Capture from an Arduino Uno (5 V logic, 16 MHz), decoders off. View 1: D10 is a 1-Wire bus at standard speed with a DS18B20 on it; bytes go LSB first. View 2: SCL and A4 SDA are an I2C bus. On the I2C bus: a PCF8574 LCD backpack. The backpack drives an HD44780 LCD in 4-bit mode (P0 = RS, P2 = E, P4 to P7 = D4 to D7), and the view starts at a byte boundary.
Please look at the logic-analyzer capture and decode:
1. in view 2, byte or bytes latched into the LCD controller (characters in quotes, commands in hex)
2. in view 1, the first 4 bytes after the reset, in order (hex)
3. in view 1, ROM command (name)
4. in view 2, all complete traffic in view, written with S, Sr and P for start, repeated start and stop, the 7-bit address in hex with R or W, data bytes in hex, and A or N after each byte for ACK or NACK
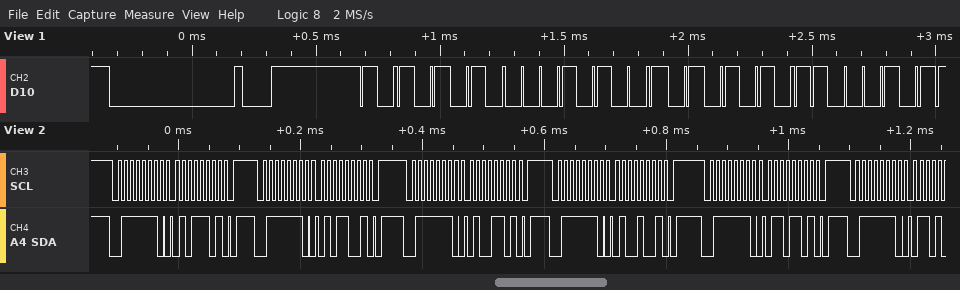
'T'
55 28 55 A3
Match ROM
S 3FW A 5D A P S 3FW A 59 A P S 3FW A 4D A P S 3FW A 49 A P S 3FW A 6D A P S 3FW A
